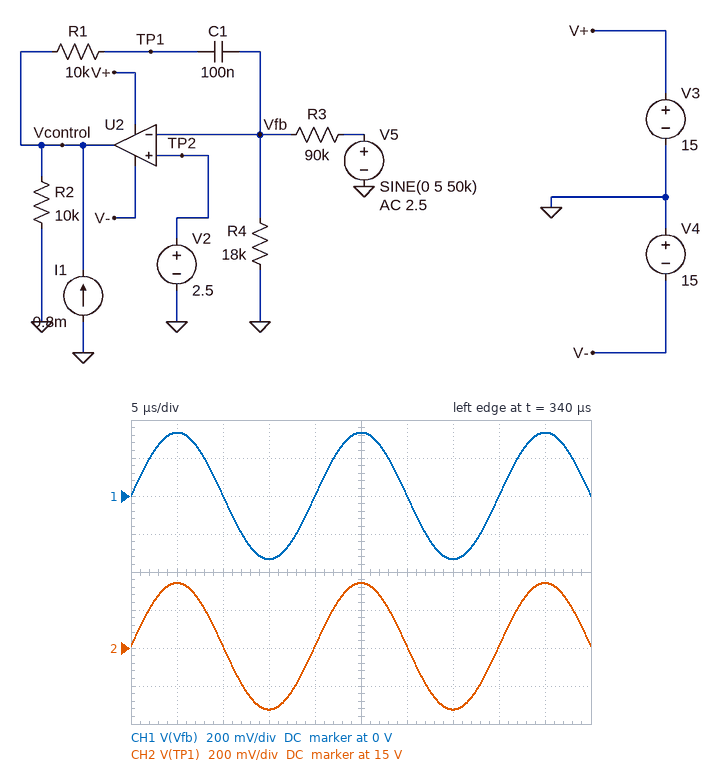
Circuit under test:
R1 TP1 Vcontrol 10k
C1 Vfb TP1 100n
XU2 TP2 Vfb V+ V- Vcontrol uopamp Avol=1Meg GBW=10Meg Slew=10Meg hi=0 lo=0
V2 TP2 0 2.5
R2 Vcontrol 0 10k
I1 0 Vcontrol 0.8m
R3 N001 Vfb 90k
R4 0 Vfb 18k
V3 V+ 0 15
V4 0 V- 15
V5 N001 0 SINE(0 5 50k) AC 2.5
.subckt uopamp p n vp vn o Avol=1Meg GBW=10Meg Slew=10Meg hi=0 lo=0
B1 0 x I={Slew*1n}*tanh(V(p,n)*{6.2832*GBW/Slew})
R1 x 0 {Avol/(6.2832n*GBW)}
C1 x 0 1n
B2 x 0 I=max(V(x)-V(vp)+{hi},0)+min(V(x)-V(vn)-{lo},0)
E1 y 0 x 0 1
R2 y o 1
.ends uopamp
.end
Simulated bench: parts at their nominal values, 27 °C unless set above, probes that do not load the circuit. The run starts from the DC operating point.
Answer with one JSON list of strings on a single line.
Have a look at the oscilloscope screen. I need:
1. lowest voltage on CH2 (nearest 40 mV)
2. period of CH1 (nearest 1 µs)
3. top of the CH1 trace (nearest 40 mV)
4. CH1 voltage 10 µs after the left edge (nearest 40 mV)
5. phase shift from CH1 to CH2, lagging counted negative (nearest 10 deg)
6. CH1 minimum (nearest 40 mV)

["14.68 V", "20 µs", "320 mV", "0 V", "0 deg", "-320 mV"]
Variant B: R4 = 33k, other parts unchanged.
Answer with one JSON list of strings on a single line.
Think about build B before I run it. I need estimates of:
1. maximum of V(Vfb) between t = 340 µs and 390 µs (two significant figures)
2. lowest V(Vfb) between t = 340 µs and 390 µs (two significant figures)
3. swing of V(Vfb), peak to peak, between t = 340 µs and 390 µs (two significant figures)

["390 mV", "-390 mV", "790 mV"]
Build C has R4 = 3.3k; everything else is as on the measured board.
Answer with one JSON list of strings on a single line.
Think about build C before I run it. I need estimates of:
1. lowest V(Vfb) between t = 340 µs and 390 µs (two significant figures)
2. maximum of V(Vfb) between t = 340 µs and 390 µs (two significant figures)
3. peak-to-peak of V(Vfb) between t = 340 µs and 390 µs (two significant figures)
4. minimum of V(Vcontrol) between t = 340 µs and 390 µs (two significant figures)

["-130 mV", "130 mV", "270 mV", "15 V"]
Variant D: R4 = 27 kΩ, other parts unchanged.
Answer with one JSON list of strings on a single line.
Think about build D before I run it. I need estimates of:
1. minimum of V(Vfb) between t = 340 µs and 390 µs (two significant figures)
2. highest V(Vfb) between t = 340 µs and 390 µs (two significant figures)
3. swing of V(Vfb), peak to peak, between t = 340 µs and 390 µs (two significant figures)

["-370 mV", "380 mV", "750 mV"]
